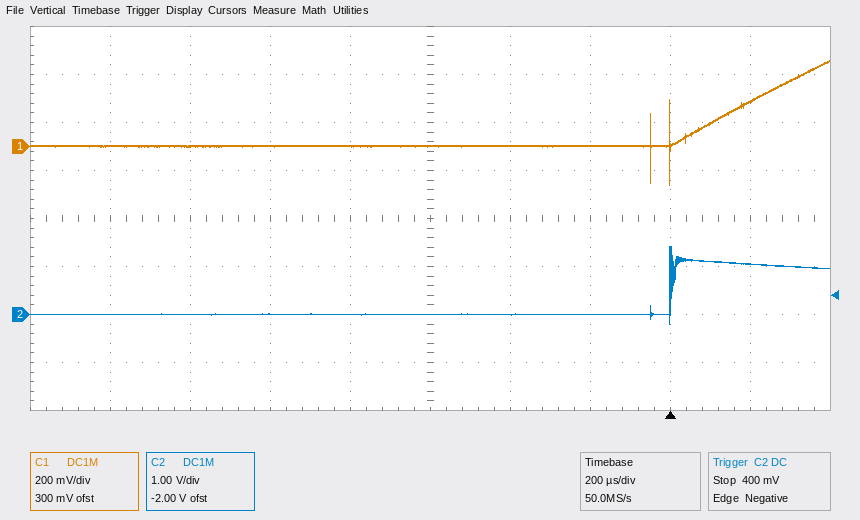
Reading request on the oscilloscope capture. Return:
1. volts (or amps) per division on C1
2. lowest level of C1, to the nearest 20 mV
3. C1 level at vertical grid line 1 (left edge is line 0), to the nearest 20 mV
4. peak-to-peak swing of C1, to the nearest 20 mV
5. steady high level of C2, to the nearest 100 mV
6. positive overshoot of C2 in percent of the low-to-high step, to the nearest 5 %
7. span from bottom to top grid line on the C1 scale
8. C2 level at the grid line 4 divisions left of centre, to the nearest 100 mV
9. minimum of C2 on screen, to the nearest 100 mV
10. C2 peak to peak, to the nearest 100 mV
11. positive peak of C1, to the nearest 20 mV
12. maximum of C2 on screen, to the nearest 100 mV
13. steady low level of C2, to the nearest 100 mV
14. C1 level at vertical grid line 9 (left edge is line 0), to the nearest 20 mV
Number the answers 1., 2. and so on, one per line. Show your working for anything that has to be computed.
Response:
1. 200 mV
2. -160 mV
3. 0 mV
4. 360 mV − (-160 mV) = 520 mV
5. 1.0 V
6. 35 %
7. 1.6 V
8. 0.0 V
9. -200 mV
10. 1.4 V − (-200 mV) = 1.6 V
11. 360 mV
12. 1.4 V
13. 0.0 V
14. 180 mV
